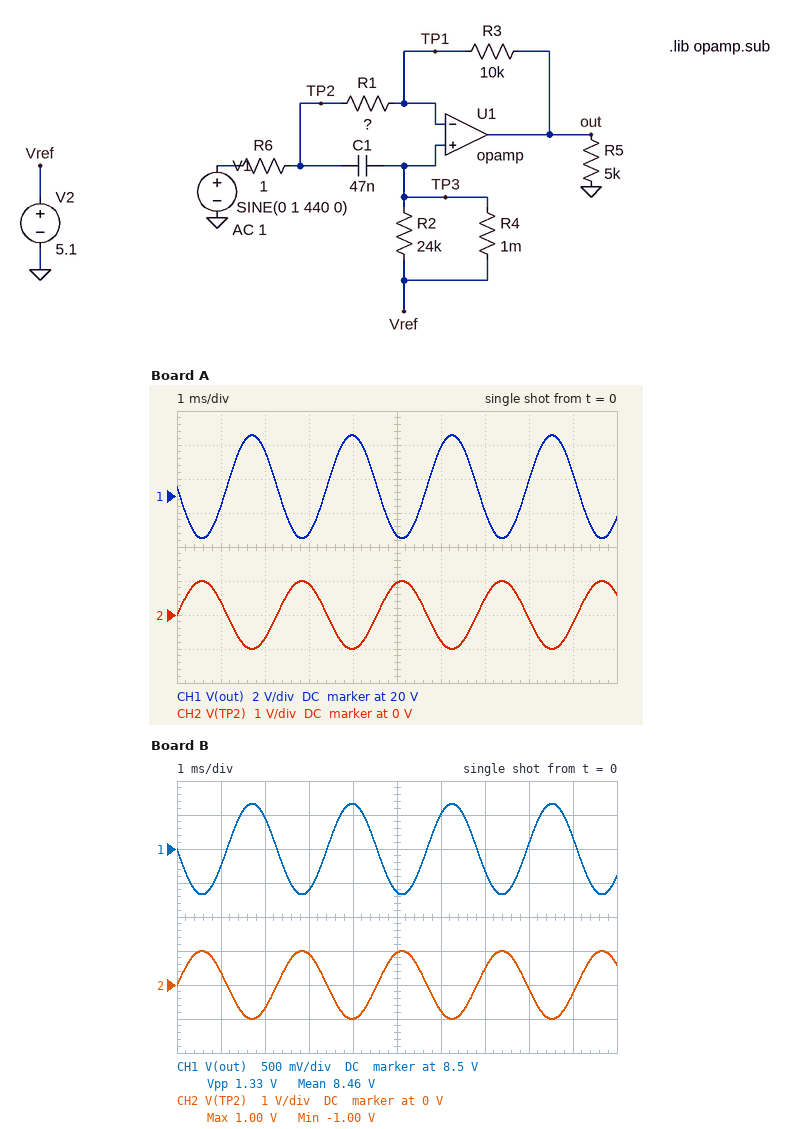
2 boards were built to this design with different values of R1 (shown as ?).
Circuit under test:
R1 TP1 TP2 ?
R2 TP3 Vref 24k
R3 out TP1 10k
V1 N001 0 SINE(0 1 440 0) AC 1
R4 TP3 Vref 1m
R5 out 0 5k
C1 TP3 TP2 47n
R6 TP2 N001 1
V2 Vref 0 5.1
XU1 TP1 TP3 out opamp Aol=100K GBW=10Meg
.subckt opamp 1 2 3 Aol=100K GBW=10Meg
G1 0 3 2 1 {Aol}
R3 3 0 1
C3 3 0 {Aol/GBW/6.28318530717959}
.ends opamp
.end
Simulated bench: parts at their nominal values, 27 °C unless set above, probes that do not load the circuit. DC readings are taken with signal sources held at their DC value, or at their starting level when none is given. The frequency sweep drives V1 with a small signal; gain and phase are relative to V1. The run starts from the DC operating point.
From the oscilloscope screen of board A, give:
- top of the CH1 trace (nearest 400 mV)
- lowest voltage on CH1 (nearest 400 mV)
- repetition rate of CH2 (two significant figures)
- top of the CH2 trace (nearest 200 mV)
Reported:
23.6 V
17.6 V
440 Hz
1.0 V
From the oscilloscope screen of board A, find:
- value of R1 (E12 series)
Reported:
3.3 kΩ
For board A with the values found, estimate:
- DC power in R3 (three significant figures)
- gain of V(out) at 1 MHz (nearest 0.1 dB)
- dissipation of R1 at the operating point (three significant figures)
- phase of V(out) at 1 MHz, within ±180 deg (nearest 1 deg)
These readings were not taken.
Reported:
23.9 mW
8.6 dB
7.88 mW
142 deg
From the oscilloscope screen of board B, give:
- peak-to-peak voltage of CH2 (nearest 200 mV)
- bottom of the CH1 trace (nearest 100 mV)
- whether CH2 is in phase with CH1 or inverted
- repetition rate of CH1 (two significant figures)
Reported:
2.0 V
7.8 V
inverted
440 Hz
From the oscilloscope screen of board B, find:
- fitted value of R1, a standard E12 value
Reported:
15 kΩ
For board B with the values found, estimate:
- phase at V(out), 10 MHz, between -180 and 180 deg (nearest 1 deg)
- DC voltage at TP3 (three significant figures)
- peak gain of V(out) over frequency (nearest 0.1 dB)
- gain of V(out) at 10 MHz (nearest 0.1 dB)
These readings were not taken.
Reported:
49 deg
5.10 V
-3.5 dB
-19.2 dB
